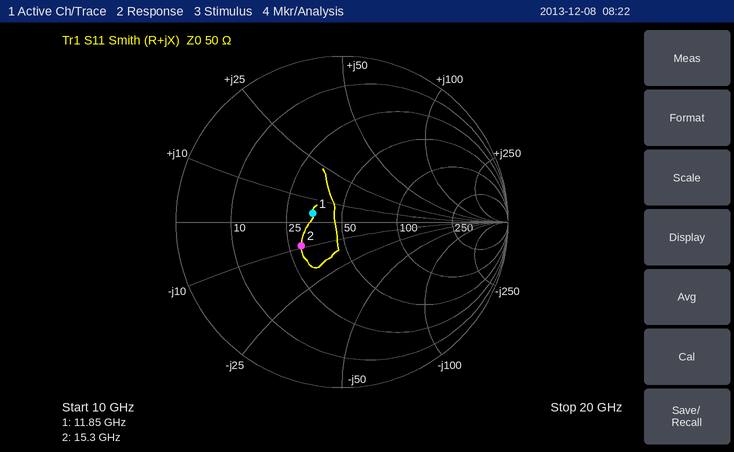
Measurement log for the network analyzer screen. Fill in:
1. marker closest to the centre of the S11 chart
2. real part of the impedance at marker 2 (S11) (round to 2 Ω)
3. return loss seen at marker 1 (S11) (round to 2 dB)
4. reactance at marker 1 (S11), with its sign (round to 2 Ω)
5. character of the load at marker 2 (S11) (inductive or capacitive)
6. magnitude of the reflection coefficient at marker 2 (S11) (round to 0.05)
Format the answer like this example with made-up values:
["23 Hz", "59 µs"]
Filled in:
["marker 1", "30 Ω", "14 dB", "+4 Ω", "capacitive", "0.30"]
